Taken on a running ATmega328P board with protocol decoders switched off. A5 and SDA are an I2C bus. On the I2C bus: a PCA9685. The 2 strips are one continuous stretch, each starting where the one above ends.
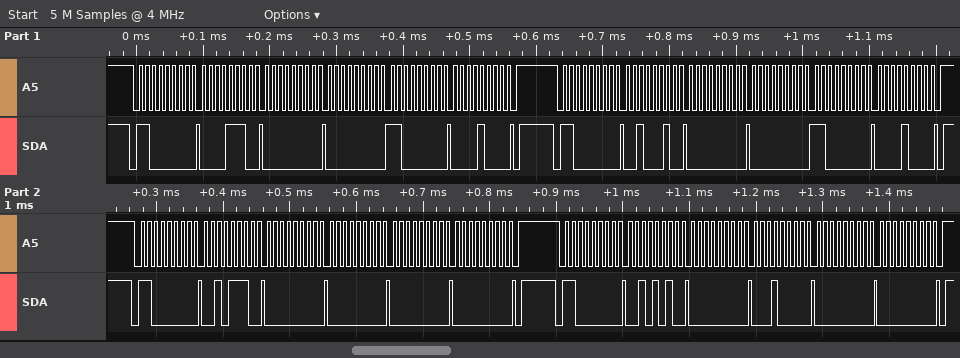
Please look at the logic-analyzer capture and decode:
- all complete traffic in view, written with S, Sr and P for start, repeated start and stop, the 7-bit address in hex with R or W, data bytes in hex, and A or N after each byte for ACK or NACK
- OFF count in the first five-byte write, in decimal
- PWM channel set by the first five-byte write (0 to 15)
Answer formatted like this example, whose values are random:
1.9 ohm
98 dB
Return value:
S 60W A 0E A 00 A 00 A C0 A 08 A P S 60W A 22 A 00 A 00 A C0 A 08 A P S 60W A 2E A 00 A 00 A 00 A 00 A P S 60W A 2A A 00 A 10 A 00 A 00 A P
2240
2
